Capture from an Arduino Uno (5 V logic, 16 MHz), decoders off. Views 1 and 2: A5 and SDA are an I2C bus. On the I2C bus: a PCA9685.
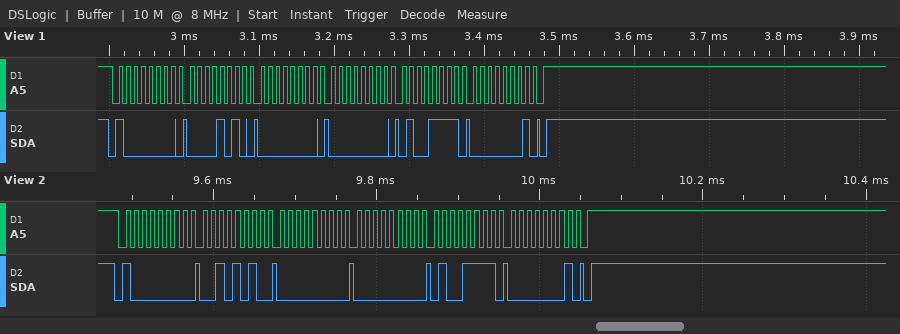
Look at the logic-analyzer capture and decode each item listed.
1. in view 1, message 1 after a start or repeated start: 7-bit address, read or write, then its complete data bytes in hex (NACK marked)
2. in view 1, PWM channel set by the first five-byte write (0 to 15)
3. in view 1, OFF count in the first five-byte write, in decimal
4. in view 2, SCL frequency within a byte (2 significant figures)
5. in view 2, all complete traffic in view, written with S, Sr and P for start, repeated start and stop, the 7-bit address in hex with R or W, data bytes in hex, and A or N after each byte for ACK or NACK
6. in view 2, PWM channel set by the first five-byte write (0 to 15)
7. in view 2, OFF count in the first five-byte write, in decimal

0x40 write: 0A 00 00 4F 01
1
335
100 kHz
S 40W A 2A A 00 A 00 A 4F A 01 A P
9
335
